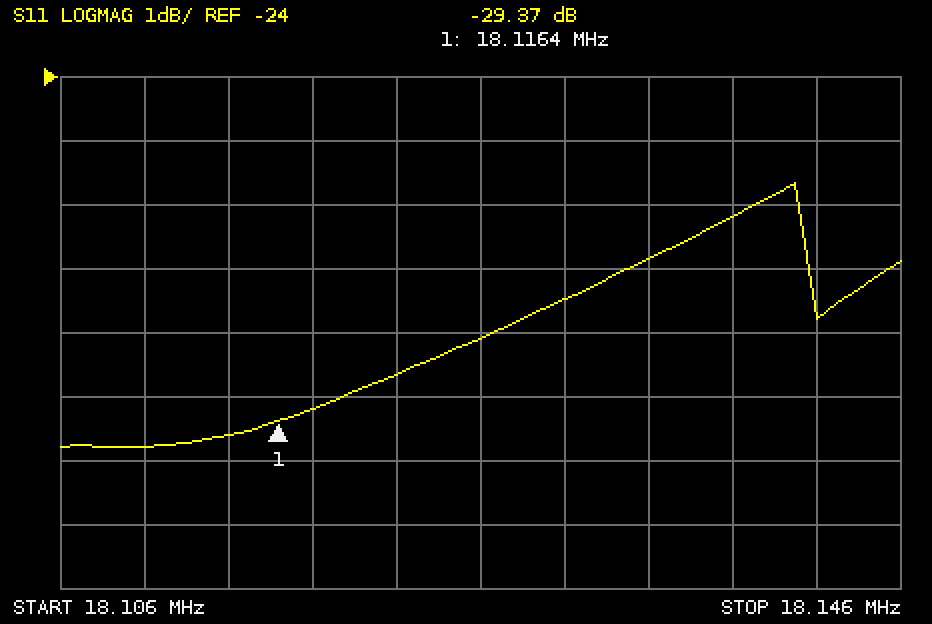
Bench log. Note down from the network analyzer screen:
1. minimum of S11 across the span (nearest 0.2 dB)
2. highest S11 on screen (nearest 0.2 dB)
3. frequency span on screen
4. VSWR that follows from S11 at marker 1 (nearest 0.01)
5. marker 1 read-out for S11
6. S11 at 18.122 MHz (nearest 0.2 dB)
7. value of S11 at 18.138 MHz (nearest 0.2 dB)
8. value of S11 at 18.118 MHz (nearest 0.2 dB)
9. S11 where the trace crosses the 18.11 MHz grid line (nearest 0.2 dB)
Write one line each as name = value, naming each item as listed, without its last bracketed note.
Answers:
minimum of S11 across the span = -29.8 dB
highest S11 on screen = -25.6 dB
frequency span on screen = 40 kHz
VSWR that follows from S11 at marker 1 = 1.07
marker 1 read-out for S11 = -29.37 dB
S11 at 18.122 MHz = -28.6 dB
value of S11 at 18.138 MHz = -26.2 dB
value of S11 at 18.118 MHz = -29.2 dB
S11 where the trace crosses the 18.11 MHz grid line = -29.8 dB
